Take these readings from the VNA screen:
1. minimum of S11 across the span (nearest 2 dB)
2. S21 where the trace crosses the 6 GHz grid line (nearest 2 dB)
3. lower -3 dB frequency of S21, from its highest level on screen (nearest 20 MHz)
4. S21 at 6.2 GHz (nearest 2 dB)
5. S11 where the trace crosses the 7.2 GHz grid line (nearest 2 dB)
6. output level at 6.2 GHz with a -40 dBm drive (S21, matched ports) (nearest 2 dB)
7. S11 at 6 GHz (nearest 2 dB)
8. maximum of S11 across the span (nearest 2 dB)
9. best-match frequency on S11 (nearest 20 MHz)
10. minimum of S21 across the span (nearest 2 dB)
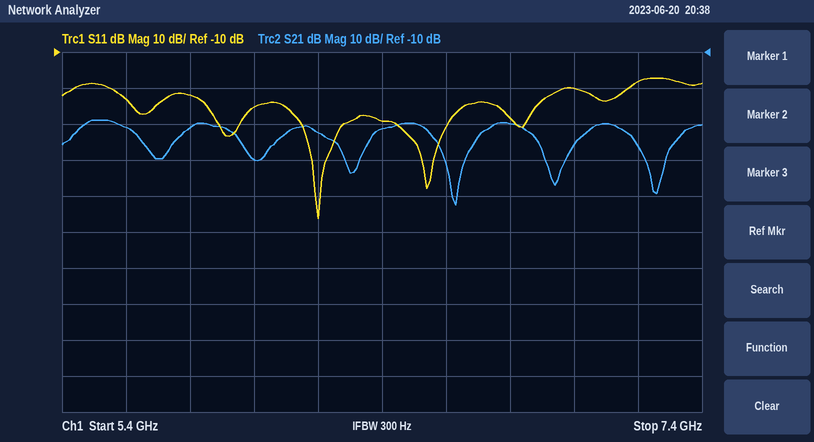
-56 dB
-40 dB
5.44 GHz
-32 dB
-18 dB
-72 dBm
-26 dB
-18 dB
6.20 GHz
-52 dB
